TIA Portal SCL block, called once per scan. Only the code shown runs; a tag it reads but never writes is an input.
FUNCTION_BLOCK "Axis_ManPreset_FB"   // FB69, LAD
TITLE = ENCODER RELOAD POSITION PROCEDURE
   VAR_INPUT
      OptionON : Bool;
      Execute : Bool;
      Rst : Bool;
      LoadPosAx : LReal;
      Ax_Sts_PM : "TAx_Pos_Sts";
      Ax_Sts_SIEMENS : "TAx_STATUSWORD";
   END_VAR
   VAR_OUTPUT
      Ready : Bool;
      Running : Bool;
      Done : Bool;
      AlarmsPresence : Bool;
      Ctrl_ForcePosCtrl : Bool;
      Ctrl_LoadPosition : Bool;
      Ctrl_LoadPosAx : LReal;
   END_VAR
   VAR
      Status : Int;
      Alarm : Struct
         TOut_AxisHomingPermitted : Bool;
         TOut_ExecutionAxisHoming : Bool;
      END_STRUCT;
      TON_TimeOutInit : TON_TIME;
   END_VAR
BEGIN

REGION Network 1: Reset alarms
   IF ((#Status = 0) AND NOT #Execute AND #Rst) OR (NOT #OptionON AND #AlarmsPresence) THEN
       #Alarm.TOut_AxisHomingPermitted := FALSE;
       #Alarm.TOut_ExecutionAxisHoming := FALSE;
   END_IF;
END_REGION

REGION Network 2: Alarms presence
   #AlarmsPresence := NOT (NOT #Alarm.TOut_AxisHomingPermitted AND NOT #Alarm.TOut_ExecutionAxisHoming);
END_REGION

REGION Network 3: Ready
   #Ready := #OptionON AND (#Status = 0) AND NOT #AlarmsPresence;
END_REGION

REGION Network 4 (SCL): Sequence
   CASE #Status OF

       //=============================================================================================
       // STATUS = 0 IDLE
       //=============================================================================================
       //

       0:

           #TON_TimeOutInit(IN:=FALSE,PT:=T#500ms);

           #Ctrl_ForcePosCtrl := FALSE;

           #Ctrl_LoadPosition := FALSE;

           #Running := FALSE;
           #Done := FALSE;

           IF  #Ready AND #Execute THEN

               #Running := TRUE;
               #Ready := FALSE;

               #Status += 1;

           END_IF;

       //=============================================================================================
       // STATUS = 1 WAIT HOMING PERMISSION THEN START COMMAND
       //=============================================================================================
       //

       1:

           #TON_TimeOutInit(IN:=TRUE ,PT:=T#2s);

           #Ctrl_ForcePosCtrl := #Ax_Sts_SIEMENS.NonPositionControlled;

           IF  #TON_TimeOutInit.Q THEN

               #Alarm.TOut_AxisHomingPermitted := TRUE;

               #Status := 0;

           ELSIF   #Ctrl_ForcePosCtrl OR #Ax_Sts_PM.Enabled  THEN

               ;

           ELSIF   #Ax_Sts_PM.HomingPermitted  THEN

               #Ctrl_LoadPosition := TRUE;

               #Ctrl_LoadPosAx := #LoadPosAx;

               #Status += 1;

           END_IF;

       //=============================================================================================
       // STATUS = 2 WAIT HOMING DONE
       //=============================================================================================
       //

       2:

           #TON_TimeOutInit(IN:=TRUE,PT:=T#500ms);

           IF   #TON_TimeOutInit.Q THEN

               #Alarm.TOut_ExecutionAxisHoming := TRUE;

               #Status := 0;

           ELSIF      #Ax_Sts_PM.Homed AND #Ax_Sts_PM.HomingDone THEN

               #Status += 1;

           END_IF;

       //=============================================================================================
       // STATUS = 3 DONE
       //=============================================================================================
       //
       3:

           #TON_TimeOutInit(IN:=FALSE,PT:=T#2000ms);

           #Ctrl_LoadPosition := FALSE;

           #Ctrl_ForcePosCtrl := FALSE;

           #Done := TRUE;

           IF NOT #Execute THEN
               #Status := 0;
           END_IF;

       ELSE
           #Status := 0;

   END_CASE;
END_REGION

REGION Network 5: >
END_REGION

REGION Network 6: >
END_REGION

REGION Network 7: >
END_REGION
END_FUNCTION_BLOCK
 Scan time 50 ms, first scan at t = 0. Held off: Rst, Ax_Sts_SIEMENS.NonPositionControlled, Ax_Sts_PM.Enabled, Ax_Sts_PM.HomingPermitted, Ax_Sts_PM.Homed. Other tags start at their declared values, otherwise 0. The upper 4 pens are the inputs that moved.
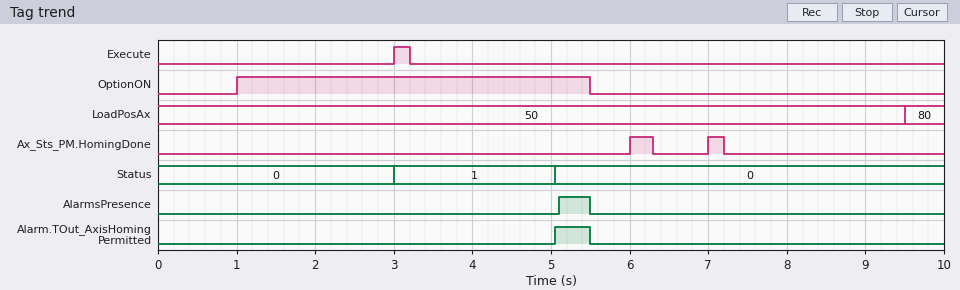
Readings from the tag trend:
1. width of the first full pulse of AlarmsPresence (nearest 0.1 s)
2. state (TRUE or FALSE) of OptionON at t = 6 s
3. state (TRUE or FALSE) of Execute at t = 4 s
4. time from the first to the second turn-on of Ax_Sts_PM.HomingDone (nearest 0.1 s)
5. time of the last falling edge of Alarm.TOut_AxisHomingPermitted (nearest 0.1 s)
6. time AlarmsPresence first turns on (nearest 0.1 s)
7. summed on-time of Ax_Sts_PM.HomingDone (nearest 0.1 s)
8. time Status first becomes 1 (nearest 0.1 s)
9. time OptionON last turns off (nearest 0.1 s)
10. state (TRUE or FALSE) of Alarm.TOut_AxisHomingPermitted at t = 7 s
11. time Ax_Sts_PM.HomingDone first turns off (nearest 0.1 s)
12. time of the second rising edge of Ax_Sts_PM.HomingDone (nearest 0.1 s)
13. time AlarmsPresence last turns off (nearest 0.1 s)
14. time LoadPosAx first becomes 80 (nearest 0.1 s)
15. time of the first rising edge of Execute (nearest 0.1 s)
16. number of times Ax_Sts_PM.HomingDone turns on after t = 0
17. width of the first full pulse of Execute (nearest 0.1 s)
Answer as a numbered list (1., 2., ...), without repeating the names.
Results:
1. 0.4 s
2. FALSE
3. FALSE
4. 1.0 s
5. 5.5 s
6. 5.1 s
7. 0.5 s
8. 3.0 s
9. 5.5 s
10. FALSE
11. 6.3 s
12. 7.0 s
13. 5.5 s
14. 9.5 s
15. 3.0 s
16. 2
17. 0.2 s
